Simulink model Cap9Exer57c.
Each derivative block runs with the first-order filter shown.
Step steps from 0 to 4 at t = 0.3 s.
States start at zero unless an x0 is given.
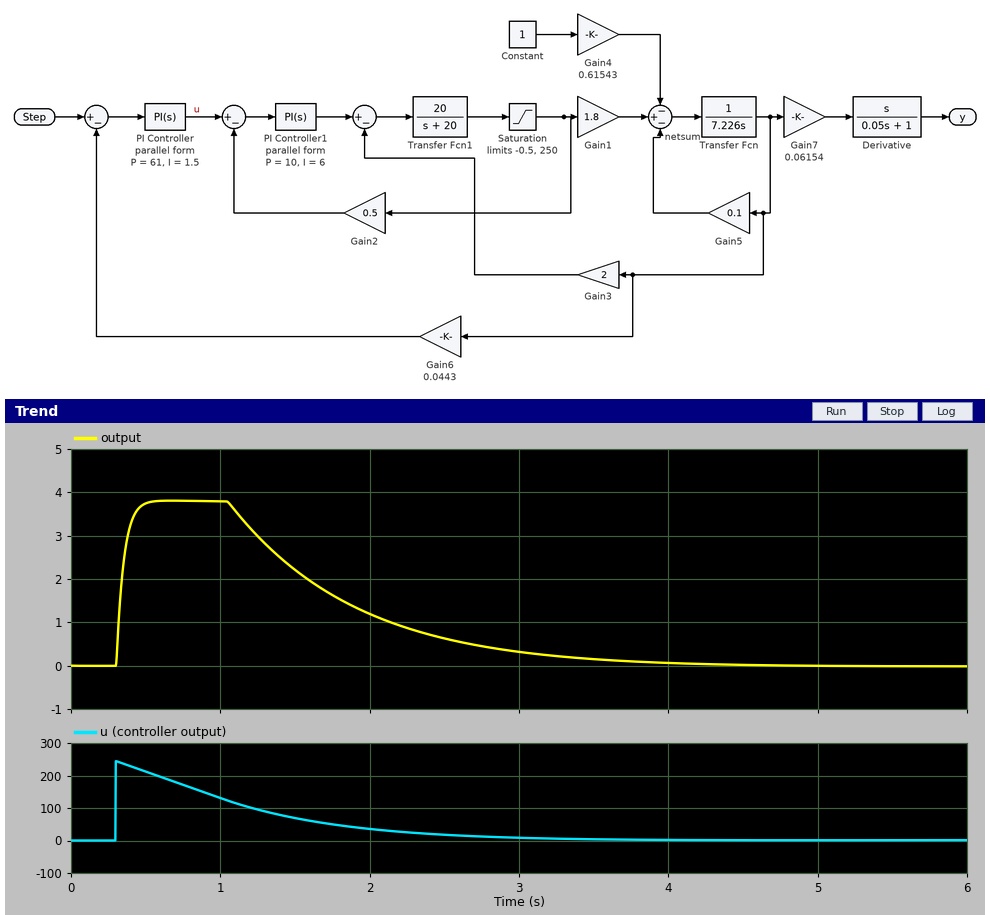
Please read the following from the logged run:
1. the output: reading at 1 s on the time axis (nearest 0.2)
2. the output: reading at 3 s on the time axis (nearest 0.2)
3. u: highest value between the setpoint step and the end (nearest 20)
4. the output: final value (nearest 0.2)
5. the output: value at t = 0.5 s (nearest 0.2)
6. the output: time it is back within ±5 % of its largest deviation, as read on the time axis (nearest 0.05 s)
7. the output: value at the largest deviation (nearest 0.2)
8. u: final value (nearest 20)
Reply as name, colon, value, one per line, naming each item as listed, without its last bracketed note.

the output: reading at 1 s on the time axis: 3.8
the output: reading at 3 s on the time axis: 0.4
u: highest value between the setpoint step and the end: 240
the output: final value: 0.0
the output: value at t = 0.5 s: 3.8
the output: time it is back within ±5 % of its largest deviation, as read on the time axis: 3.35 s
the output: value at the largest deviation: 3.8
u: final value: 0
